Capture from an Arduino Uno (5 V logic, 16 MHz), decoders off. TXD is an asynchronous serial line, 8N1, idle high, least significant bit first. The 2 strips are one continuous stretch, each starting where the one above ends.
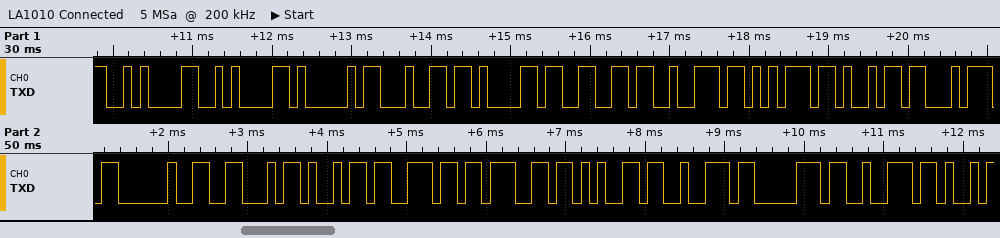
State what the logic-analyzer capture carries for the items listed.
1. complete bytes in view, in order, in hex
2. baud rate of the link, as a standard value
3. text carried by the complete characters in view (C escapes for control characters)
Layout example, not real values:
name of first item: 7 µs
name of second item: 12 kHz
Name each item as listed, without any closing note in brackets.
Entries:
complete bytes in view, in order, in hex: 0A 0A 41 64 61 66 72 75 69 74 20 46 69 6E 67 65 72 70 72
baud rate of the link, as a standard value: 9600 baud
text carried by the complete characters in view: "\n\nAdafruit Fingerpr"
